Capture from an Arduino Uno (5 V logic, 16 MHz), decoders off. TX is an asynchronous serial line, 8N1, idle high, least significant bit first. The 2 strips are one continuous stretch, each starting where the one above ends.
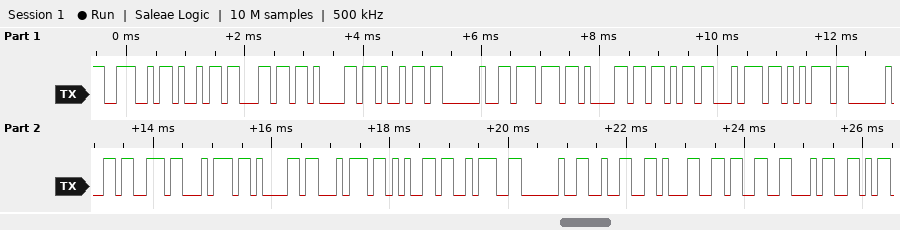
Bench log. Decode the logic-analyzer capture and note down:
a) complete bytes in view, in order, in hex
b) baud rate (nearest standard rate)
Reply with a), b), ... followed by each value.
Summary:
a) 0x4E 0x69 0x6C 0x61 0x69 0x20 0x77 0x61 0x6B 0x74 0x75 0x20 0x73 0x74 0x61 0x74 0x65 0x3A 0x20 0x32 0x31 0x33 0x34
b) 9600 baud
